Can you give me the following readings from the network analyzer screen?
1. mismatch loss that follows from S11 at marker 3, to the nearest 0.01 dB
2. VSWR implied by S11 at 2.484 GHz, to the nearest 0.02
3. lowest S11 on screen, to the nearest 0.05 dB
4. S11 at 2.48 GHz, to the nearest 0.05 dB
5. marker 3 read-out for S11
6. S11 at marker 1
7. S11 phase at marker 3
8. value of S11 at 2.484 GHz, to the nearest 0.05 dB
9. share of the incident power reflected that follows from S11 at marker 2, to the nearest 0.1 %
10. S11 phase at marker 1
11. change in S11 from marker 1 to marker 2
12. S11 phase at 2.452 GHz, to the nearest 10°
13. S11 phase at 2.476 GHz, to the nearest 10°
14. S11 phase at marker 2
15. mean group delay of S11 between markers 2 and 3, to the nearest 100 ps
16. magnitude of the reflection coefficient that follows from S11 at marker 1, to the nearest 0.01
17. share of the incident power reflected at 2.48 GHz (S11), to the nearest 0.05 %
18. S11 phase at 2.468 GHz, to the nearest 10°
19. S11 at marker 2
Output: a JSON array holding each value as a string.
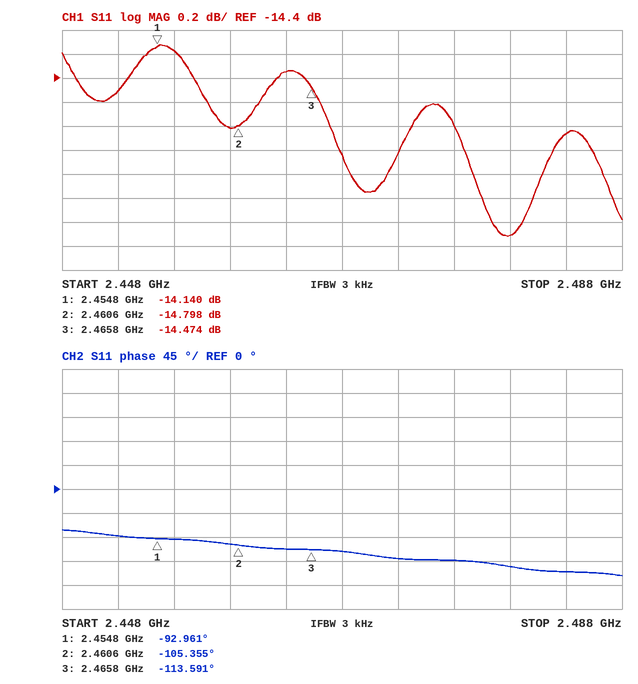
["0.16 dB", "1.44", "-15.70 dB", "-15.70 dB", "-14.474 dB", "-14.140 dB", "-113.591°", "-14.85 dB", "3.3 %", "-92.961°", "-0.658 dB", "-90°", "-130°", "-105.355°", "4.4 ns", "0.20", "2.70 %", "-120°", "-14.798 dB"]
